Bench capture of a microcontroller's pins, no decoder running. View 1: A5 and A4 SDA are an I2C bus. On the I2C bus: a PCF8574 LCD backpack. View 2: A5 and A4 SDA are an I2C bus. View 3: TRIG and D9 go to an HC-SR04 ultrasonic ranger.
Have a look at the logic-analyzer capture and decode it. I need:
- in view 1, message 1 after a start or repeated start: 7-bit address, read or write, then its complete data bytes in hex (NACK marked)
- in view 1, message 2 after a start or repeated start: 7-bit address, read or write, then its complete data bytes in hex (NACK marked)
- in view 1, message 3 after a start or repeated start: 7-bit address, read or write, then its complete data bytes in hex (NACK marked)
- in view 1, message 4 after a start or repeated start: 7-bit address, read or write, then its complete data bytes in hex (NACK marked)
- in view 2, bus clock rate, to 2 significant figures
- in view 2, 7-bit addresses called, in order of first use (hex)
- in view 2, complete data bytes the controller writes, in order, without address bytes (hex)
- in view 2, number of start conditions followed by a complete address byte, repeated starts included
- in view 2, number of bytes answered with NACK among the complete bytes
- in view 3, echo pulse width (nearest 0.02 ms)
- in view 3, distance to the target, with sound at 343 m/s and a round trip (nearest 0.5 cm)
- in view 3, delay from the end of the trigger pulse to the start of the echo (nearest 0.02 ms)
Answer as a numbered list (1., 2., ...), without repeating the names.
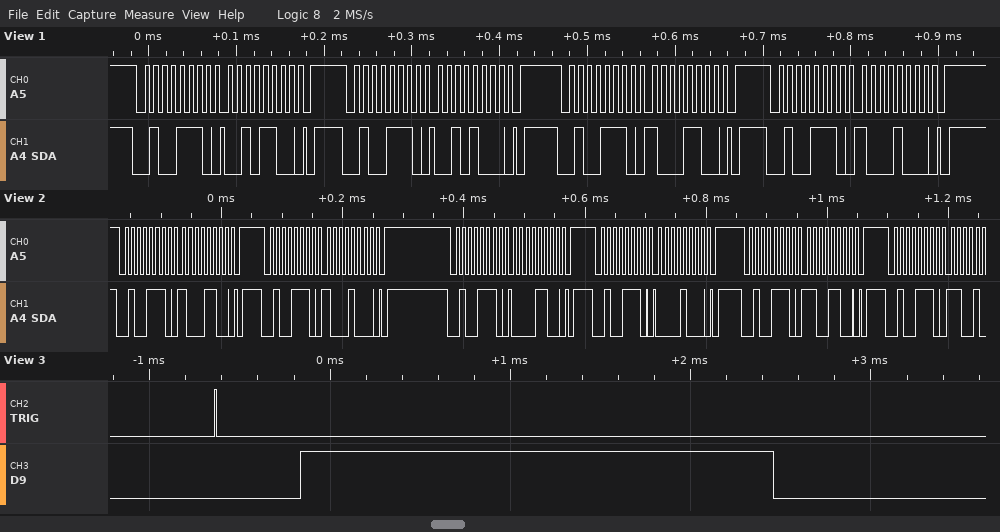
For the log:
1. 0x27 write: 2C
2. 0x27 write: 28
3. 0x27 write: 8C
4. 0x27 write: 88
5. 100 kHz
6. 0x27
7. 8C 88 0C 08 CC
8. 6
9. 0
10. 2.62 ms
11. 45 cm
12. 0.46 ms
